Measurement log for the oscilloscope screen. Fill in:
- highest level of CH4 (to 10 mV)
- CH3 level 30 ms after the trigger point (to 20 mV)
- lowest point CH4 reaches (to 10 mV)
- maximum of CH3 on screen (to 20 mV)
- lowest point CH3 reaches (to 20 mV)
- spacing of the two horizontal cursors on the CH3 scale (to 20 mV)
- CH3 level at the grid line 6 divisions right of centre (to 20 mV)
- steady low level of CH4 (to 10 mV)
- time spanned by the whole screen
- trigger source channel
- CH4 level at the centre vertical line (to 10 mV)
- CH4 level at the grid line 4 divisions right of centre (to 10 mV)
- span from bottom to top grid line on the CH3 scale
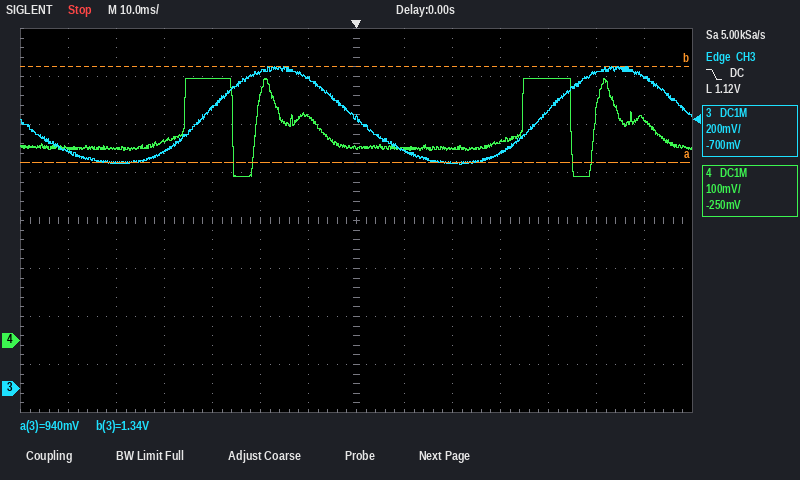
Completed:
550 mV
980 mV
340 mV
1.34 V
940 mV
400 mV
1.30 V
400 mV
140 ms
CH3
400 mV
550 mV
1.6 V
